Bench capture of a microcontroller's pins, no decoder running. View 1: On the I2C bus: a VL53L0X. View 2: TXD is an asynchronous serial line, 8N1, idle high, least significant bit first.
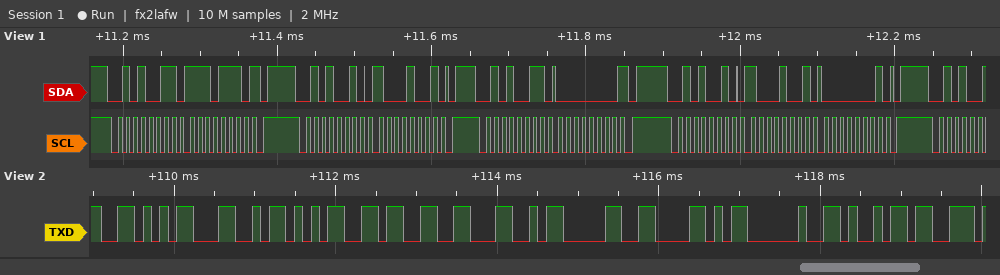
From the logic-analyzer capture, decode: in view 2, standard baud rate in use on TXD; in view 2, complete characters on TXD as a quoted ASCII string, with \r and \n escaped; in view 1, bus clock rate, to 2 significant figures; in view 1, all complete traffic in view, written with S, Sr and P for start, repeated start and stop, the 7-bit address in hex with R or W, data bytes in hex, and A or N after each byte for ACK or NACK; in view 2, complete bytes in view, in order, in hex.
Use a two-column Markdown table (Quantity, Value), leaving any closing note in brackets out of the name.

| Quantity | Value |
|---|---|
| in view 2, standard baud rate in use on TXD | 9600 baud |
| in view 2, complete characters on TXD as a quoted ASCII string, with \r and \n escaped | "VL53L0X i" |
| in view 1, bus clock rate, to 2 significant figures | 100 kHz |
| in view 1, all complete traffic in view, written with S, Sr and P for start, repeated start and stop, the 7-bit address in hex with R or W, data bytes in hex, and A or N after each byte for ACK or NACK | S 29R A EE N P S 29W A 89 A P S 29R A 00 N P S 29W A 89 A 01 A P |
| in view 2, complete bytes in view, in order, in hex | 0x56 0x4C 0x35 0x33 0x4C 0x30 0x58 0x20 0x69 |
